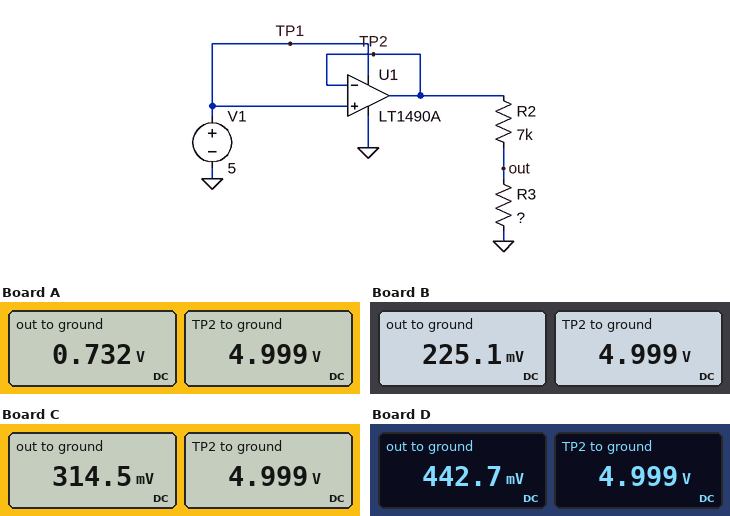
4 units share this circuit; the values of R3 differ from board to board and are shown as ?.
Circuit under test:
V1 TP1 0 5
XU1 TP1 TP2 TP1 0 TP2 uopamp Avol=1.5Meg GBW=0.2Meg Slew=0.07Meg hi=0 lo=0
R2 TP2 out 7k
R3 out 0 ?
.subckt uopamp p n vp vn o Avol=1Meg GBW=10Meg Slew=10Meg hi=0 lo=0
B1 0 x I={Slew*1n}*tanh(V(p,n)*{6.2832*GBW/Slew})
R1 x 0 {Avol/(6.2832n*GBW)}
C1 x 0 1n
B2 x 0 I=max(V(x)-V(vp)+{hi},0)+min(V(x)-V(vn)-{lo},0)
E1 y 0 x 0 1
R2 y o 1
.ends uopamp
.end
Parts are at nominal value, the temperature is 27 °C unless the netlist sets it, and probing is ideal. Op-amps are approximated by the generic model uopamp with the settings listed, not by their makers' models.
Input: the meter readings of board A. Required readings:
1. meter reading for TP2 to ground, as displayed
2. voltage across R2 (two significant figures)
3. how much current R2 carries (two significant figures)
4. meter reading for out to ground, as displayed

4.999 V
4.3 V
610 µA
0.732 V
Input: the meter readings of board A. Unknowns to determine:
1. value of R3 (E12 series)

1.2 kΩ
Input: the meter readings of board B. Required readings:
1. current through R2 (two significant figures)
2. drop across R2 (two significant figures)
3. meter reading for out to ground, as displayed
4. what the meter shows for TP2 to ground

680 µA
4.8 V
225.1 mV
4.999 V
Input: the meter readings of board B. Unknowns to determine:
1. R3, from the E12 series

330 Ω
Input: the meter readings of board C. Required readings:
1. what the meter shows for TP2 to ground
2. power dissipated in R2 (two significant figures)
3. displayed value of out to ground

4.999 V
3.1 mW
314.5 mV
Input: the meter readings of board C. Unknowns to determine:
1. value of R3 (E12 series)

470 Ω
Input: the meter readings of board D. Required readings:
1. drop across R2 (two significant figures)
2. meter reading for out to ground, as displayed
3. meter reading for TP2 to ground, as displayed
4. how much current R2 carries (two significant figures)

4.6 V
442.7 mV
4.999 V
650 µA
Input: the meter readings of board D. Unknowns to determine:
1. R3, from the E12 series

680 Ω
